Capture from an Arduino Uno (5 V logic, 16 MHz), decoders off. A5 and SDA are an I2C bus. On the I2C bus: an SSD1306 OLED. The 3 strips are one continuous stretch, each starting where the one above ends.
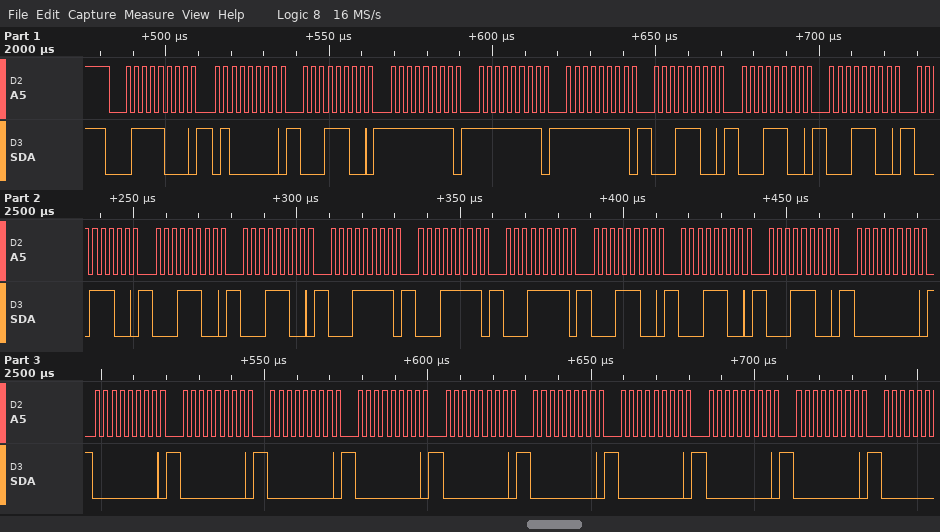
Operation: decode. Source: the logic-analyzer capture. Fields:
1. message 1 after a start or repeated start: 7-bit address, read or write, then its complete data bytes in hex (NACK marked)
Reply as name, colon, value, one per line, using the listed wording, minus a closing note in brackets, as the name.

message 1 after a start or repeated start: 7-bit address, read or write, then its complete data bytes in hex: 0x3C write: 40 1C FF FF FF 1C 1C 1C 1C 1C 1C 1F 1F 1F 1C 1C 1C 00 00 00 00 00 00 00 00 00 00
